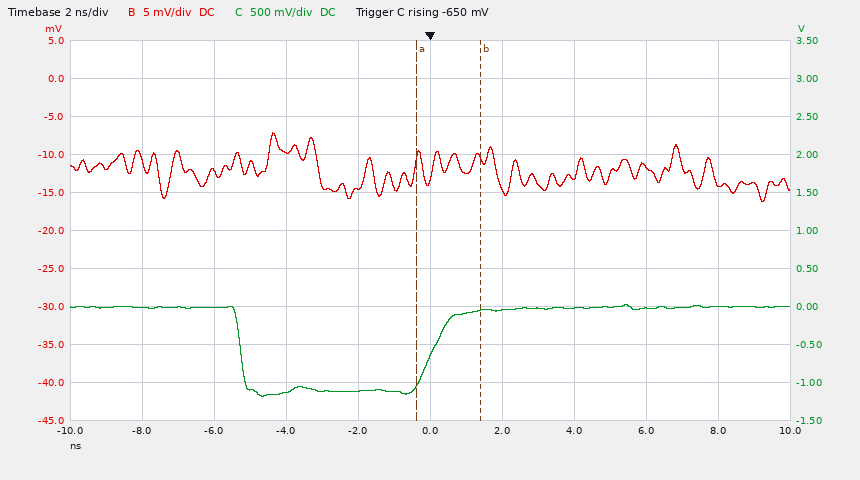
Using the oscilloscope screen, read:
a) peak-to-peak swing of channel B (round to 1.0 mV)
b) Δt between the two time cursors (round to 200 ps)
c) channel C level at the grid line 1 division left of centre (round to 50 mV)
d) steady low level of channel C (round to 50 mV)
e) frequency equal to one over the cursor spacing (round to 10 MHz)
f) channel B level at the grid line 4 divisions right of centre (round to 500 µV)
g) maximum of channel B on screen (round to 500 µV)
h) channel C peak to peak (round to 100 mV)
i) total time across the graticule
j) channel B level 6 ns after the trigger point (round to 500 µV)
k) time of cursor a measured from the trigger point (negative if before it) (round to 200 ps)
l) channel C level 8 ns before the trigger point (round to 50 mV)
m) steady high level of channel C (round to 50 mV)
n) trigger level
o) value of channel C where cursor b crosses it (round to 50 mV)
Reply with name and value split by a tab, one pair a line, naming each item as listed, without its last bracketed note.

peak-to-peak swing of channel B	9.0 mV
Δt between the two time cursors	1.8 ns
channel C level at the grid line 1 division left of centre	-1.10 V
steady low level of channel C	-1.10 V
frequency equal to one over the cursor spacing	560 MHz
channel B level at the grid line 4 divisions right of centre	-14.0 mV
maximum of channel B on screen	-7.0 mV
channel C peak to peak	1.20 V
total time across the graticule	20 ns
channel B level 6 ns after the trigger point	-11.5 mV
time of cursor a measured from the trigger point (negative if before it)	-400 ps
channel C level 8 ns before the trigger point	0 mV
steady high level of channel C	0 mV
trigger level	-650 mV
value of channel C where cursor b crosses it	-50 mV
